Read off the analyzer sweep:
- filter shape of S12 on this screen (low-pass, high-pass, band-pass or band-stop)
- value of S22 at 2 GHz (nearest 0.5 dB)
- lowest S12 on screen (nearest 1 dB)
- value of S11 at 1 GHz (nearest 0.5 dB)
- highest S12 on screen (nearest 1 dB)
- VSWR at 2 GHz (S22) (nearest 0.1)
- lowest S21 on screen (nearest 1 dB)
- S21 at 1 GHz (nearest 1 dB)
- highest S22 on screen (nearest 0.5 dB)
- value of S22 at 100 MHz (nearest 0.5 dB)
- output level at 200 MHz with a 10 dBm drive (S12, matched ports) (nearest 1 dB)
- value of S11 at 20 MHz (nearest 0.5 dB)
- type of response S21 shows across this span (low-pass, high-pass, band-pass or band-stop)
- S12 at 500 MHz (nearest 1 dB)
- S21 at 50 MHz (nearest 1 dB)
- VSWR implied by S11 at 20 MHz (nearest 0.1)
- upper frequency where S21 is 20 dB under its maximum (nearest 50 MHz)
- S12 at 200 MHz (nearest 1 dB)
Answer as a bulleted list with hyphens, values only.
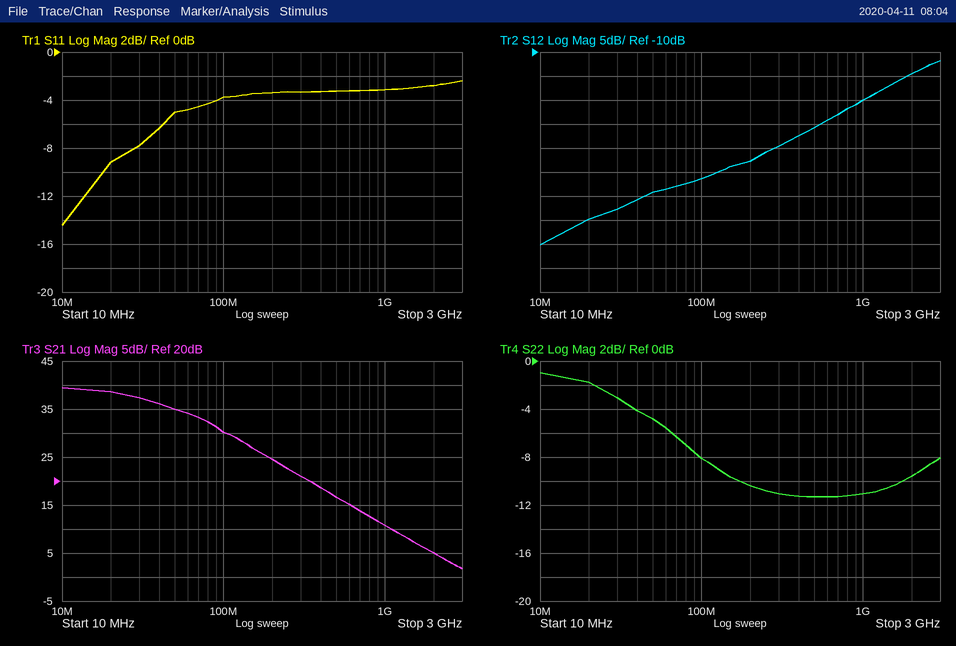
- high-pass
- -9.5 dB
- -50 dB
- -3.0 dB
- -12 dB
- 2.0
- 2 dB
- 11 dB
- -1.0 dB
- -8.0 dB
- -23 dBm
- -9.0 dB
- low-pass
- -26 dB
- 35 dB
- 2.1
- 350 MHz
- -33 dB
